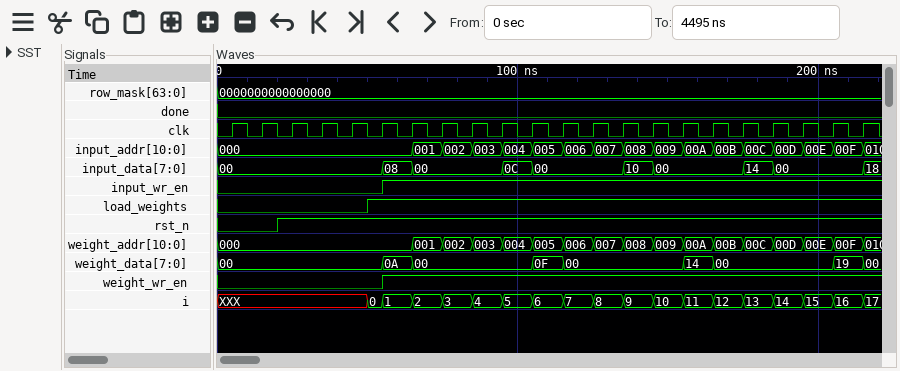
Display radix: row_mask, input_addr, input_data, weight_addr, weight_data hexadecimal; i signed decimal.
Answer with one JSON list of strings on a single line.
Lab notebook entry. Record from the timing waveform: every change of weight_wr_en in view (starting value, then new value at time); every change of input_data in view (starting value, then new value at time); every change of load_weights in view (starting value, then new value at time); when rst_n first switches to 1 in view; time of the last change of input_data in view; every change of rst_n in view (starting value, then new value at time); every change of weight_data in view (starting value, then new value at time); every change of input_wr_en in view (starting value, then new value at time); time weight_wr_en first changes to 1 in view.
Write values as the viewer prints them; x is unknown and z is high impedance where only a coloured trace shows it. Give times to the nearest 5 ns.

["0, 1 at 55 ns", "00, 08 at 55 ns, 00 at 65 ns, 0C at 95 ns, 00 at 105 ns, 10 at 135 ns, 00 at 145 ns, 14 at 175 ns, 00 at 185 ns, 18 at 215 ns", "0, 1 at 50 ns", "20 ns", "215 ns", "0, 1 at 20 ns", "00, 0A at 55 ns, 00 at 65 ns, 0F at 105 ns, 00 at 115 ns, 14 at 155 ns, 00 at 165 ns, 19 at 205 ns, 00 at 215 ns", "0, 1 at 55 ns", "55 ns"]
